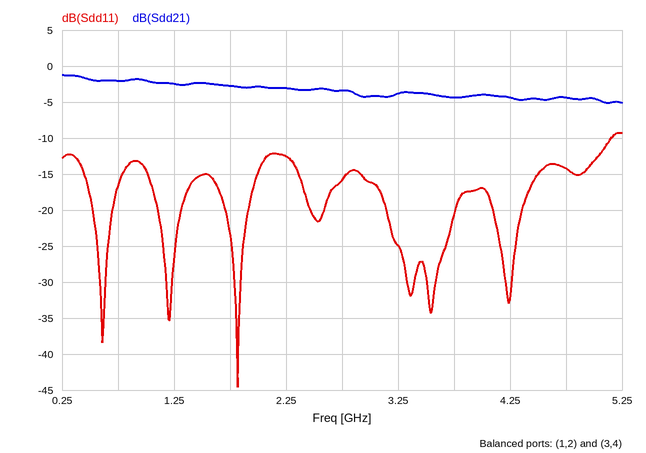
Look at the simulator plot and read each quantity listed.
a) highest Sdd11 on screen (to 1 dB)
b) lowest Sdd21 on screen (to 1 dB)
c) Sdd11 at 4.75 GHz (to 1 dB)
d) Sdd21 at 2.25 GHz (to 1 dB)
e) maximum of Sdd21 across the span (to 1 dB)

-9 dB
-5 dB
-14 dB
-3 dB
-1 dB
